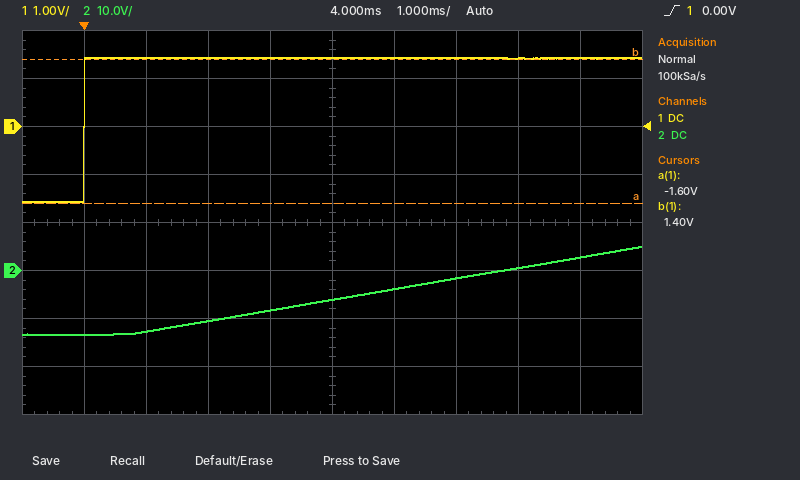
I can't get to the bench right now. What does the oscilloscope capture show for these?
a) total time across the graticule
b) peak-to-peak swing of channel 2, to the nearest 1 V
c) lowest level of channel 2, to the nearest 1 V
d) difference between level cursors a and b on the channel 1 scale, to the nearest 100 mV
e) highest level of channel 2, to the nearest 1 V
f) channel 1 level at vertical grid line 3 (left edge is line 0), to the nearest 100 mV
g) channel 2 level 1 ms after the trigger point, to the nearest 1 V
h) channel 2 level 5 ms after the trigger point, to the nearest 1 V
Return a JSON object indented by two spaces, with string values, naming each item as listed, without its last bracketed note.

{
  "total time across the graticule": "10 ms",
  "peak-to-peak swing of channel 2, to the nearest 1 V": "18 V",
  "lowest level of channel 2, to the nearest 1 V": "-13 V",
  "difference between level cursors a and b on the channel 1 scale, to the nearest 100 mV": "3.0 V",
  "highest level of channel 2, to the nearest 1 V": "5 V",
  "channel 1 level at vertical grid line 3 (left edge is line 0), to the nearest 100 mV": "1.4 V",
  "channel 2 level 1 ms after the trigger point, to the nearest 1 V": "-13 V",
  "channel 2 level 5 ms after the trigger point, to the nearest 1 V": "-4 V"
}
